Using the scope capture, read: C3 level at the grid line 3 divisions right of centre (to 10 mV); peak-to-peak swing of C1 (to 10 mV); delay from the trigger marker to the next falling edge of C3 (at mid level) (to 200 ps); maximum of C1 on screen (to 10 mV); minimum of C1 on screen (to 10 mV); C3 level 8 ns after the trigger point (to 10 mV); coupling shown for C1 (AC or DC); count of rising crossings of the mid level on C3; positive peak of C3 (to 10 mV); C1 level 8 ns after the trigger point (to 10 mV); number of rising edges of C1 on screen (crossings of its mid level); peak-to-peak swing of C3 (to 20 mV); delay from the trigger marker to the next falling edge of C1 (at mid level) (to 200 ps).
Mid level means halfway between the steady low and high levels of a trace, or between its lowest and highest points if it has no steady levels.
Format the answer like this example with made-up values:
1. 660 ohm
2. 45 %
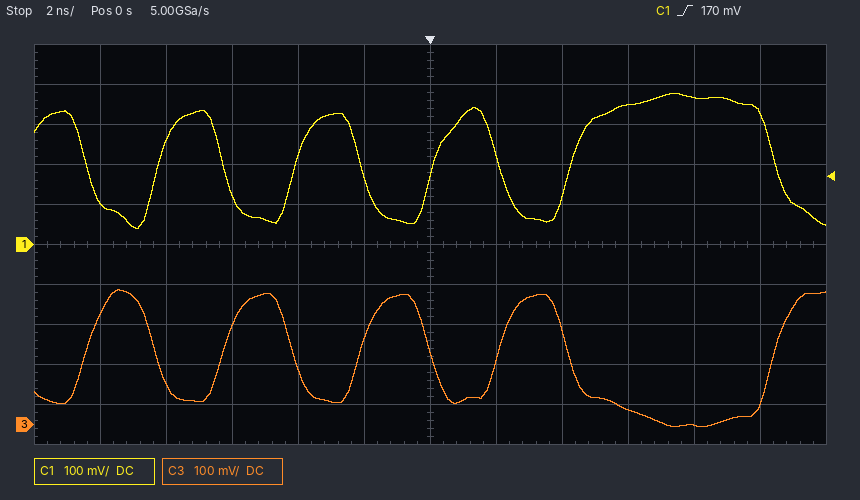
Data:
1. 40 mV
2. 340 mV
3. 4.2 ns
4. 380 mV
5. 40 mV
6. 0 mV
7. DC
8. 5
9. 340 mV
10. 370 mV
11. 4
12. 340 mV
13. 2.0 ns
